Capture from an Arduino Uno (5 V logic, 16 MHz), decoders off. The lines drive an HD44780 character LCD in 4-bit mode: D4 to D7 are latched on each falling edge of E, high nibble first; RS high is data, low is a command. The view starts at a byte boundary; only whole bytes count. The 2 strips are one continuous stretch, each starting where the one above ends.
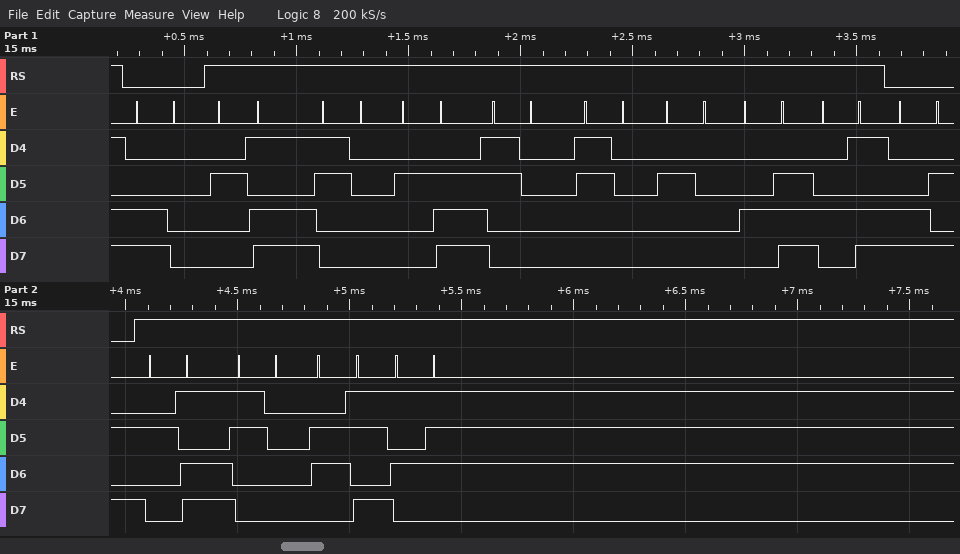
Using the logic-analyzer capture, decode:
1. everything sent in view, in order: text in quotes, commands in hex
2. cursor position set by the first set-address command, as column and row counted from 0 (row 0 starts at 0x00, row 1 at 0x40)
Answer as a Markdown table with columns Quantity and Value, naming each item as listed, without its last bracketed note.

| Quantity | Value |
|---|---|
| everything sent in view, in order: text in quotes, commands in hex | 0xC0 "-0.00 NM" 0xCA "-0kW" |
| cursor position set by the first set-address command, as column and row counted from 0 | column 0, row 1 |
